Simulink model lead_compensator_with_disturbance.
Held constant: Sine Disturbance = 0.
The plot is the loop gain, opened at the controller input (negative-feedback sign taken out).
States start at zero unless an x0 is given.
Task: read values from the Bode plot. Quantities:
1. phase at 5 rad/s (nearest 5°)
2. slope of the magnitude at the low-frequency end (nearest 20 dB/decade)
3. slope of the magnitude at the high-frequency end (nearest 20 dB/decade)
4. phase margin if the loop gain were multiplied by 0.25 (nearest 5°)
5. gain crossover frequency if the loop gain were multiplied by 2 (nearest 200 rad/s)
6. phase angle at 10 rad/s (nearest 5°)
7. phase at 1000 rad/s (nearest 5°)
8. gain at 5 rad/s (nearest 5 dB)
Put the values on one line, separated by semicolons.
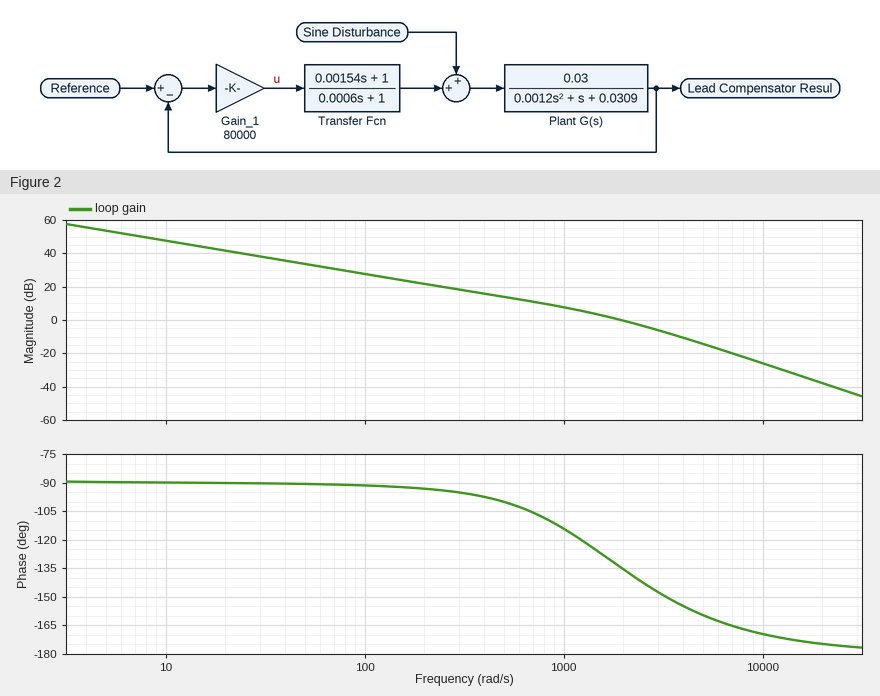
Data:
-90°; -20 dB/decade; -40 dB/decade; 75°; 3000 rad/s; -90°; -115°; 55 dB
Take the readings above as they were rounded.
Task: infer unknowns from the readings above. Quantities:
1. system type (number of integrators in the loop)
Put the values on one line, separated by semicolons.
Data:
1
